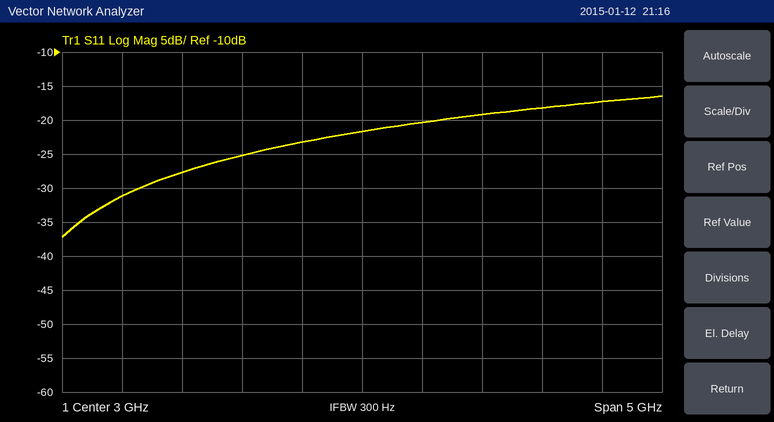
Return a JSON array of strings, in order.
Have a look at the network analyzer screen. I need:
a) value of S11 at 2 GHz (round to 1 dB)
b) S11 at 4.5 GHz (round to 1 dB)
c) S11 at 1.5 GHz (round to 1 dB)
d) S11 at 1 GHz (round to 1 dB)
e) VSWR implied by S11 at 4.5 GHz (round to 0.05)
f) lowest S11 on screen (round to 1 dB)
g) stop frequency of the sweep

["-25 dB", "-18 dB", "-28 dB", "-31 dB", "1.30", "-37 dB", "5.5 GHz"]
